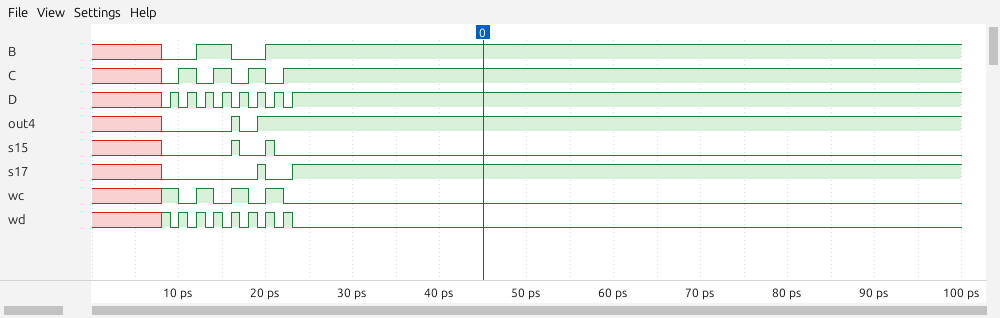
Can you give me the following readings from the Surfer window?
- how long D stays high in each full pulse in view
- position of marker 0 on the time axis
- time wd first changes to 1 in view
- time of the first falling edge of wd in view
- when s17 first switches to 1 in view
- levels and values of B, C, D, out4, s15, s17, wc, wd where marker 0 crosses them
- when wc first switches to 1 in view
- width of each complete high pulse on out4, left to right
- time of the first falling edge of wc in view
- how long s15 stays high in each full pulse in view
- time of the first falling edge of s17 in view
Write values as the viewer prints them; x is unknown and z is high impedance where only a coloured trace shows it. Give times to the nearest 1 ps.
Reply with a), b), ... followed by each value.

a) 1 ps, 1 ps, 1 ps, 1 ps, 1 ps, 1 ps, 1 ps
b) 45 ps
c) 8 ps
d) 9 ps
e) 19 ps
f) B=1, C=1, D=1, out4=1, s15=0, s17=1, wc=0, wd=0
g) 8 ps
h) 1 ps
i) 10 ps
j) 1 ps, 1 ps
k) 20 ps
